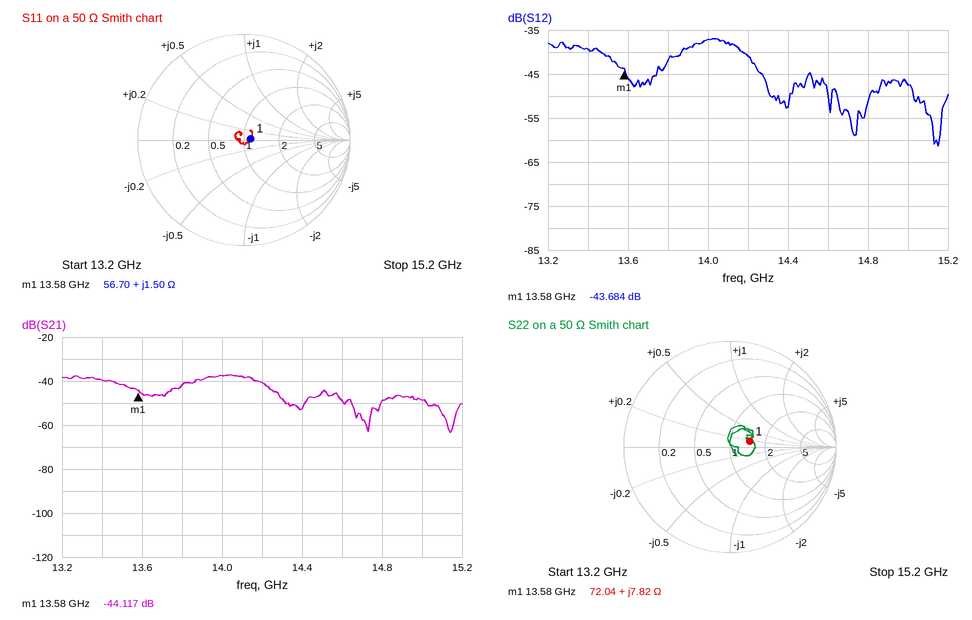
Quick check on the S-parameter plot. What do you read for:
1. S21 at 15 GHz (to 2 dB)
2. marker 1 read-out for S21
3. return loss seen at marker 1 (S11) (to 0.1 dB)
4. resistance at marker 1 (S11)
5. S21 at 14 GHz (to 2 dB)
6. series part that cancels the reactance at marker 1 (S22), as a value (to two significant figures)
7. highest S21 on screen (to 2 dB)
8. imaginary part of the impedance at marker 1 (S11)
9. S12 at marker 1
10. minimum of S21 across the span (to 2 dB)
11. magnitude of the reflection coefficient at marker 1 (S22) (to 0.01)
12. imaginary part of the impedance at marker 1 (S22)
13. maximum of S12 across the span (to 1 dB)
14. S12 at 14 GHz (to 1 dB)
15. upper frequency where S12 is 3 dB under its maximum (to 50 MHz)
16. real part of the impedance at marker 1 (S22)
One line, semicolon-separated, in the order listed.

-48 dB; -44.117 dB; 23.8 dB; 56.70 Ω; -38 dB; 1.5 pF; -38 dB; +1.50 Ω; -43.684 dB; -64 dB; 0.19; +7.82 Ω; -37 dB; -37 dB; 14.15 GHz; 72.04 Ω
